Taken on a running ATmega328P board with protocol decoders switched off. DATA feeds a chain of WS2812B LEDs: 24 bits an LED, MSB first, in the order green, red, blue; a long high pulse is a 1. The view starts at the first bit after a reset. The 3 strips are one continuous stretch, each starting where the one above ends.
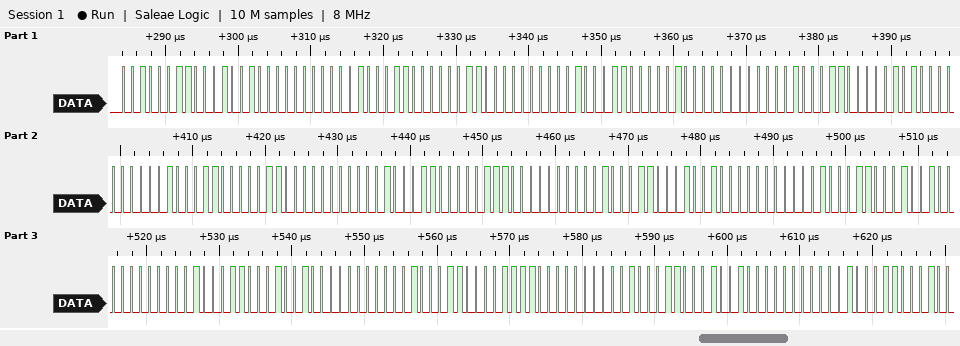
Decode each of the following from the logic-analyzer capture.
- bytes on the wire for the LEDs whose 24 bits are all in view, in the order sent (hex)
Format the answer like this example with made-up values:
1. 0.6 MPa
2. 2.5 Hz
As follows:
1. 23 12 00 23 03 00 23 04 00 23 05 00 23 06 00 23 07 00 23 12 00 23 12 00 23 12 00 23 0F 00 23 12 00
